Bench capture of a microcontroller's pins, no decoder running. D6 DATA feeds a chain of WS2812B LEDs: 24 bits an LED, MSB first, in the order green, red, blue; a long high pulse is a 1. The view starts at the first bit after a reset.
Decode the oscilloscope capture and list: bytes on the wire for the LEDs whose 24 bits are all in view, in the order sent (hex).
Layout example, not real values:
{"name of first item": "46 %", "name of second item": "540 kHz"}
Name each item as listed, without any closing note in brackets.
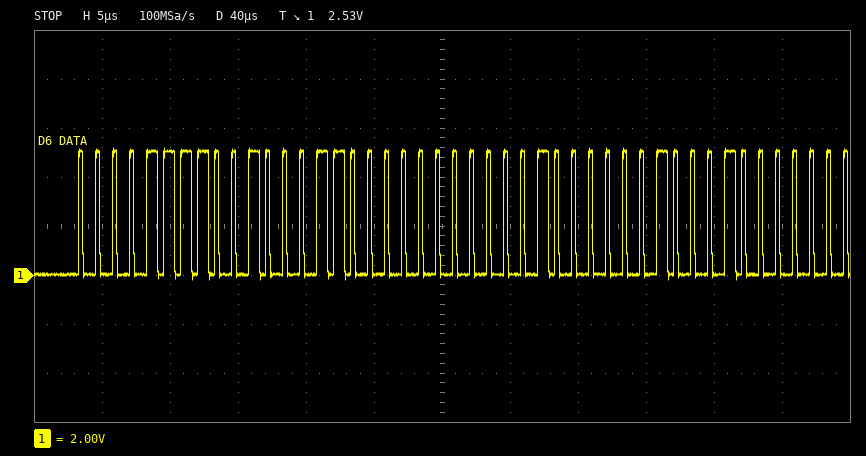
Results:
{"bytes on the wire for the LEDs whose 24 bits are all in view, in the order sent": "0F 23 00"}
